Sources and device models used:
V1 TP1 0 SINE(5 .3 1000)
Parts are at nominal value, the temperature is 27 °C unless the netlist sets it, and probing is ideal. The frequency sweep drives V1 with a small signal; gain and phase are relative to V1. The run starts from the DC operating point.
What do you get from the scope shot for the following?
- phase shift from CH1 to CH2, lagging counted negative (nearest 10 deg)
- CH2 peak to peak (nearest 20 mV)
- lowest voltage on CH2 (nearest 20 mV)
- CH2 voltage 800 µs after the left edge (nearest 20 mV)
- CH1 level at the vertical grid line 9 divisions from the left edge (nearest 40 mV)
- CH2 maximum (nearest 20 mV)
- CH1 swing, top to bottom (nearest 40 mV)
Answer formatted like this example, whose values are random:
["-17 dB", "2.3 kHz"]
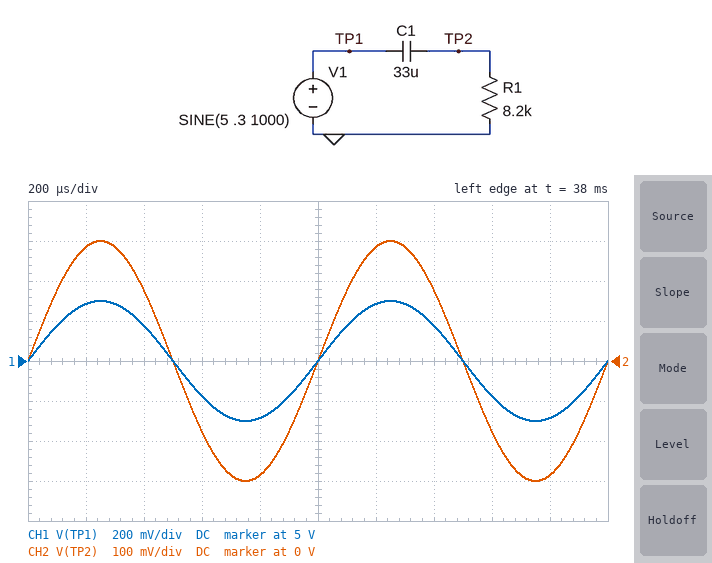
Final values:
["0 deg", "600 mV", "-300 mV", "-280 mV", "4.72 V", "300 mV", "600 mV"]
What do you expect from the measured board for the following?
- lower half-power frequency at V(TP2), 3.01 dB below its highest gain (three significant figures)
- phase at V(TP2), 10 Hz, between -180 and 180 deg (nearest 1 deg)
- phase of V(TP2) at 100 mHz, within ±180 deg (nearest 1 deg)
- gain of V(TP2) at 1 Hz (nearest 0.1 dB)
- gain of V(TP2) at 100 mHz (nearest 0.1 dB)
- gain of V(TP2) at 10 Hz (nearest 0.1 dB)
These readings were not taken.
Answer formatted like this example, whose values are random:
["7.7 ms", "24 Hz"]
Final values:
["588 mHz", "3 deg", "80 deg", "-1.3 dB", "-15.5 dB", "0 dB"]
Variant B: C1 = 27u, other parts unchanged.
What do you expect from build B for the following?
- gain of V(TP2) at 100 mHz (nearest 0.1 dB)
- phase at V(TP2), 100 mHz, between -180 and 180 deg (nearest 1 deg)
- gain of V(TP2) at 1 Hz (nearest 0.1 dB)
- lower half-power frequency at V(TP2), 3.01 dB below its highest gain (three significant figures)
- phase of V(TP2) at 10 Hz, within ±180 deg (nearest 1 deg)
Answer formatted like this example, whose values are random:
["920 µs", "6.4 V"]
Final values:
["-17.2 dB", "82 deg", "-1.8 dB", "719 mHz", "4 deg"]
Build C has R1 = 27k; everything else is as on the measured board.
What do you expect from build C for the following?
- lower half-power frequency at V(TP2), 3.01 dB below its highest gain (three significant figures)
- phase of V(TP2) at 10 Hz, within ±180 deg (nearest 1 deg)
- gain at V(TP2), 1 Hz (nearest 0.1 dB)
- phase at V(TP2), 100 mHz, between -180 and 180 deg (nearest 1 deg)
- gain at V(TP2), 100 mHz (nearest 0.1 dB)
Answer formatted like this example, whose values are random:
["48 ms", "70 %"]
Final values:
["179 mHz", "1 deg", "-0.1 dB", "61 deg", "-6.2 dB"]
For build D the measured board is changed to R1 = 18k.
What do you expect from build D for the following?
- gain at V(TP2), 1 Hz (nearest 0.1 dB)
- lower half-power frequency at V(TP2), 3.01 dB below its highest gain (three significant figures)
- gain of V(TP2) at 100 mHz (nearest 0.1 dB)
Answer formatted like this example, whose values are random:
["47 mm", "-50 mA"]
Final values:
["-0.3 dB", "268 mHz", "-9.1 dB"]
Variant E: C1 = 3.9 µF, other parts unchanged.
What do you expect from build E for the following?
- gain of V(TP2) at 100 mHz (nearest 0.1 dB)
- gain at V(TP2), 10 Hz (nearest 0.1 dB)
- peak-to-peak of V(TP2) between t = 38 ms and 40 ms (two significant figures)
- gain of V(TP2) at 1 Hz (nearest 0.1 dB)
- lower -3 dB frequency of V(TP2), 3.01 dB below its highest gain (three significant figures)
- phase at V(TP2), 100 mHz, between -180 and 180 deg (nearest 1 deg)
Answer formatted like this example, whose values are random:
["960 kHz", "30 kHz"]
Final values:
["-33.9 dB", "-1.0 dB", "600 mV", "-14.1 dB", "4.98 Hz", "89 deg"]
